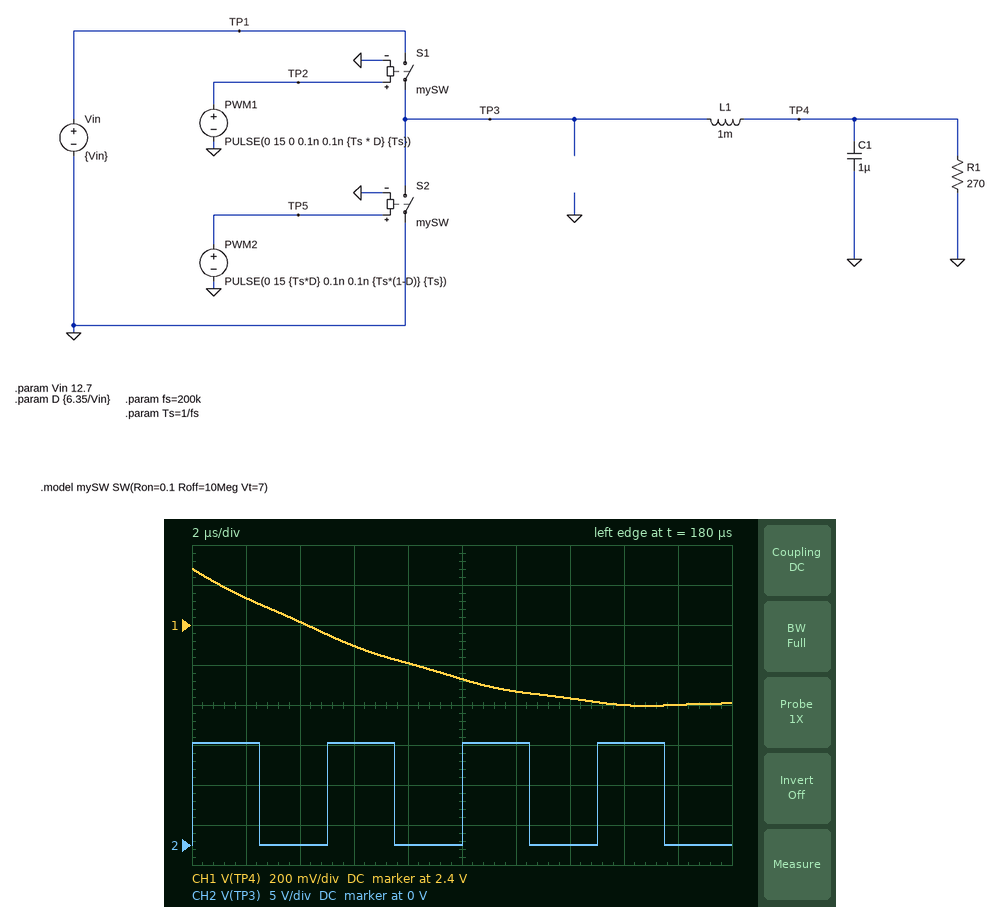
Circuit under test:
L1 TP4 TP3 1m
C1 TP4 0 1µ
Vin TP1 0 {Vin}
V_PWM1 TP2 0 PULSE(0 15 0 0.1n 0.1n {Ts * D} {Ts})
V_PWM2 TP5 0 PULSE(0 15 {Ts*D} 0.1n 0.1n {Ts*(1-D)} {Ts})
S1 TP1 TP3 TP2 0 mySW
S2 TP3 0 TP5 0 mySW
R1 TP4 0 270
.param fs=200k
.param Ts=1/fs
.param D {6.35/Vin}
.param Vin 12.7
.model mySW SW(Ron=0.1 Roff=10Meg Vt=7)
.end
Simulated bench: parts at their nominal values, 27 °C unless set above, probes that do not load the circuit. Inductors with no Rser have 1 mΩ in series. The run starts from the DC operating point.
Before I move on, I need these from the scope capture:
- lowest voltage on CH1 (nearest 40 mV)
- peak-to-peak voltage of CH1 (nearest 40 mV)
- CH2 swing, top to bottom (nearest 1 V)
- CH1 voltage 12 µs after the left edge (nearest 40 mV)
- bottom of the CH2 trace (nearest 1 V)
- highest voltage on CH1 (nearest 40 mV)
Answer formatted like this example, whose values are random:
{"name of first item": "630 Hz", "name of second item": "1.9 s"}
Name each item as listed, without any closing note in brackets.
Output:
{"lowest voltage on CH1": "2.00 V", "peak-to-peak voltage of CH1": "680 mV", "CH2 swing, top to bottom": "13 V", "CH1 voltage 12 µs after the left edge": "2.08 V", "bottom of the CH2 trace": "0 V", "highest voltage on CH1": "2.68 V"}
